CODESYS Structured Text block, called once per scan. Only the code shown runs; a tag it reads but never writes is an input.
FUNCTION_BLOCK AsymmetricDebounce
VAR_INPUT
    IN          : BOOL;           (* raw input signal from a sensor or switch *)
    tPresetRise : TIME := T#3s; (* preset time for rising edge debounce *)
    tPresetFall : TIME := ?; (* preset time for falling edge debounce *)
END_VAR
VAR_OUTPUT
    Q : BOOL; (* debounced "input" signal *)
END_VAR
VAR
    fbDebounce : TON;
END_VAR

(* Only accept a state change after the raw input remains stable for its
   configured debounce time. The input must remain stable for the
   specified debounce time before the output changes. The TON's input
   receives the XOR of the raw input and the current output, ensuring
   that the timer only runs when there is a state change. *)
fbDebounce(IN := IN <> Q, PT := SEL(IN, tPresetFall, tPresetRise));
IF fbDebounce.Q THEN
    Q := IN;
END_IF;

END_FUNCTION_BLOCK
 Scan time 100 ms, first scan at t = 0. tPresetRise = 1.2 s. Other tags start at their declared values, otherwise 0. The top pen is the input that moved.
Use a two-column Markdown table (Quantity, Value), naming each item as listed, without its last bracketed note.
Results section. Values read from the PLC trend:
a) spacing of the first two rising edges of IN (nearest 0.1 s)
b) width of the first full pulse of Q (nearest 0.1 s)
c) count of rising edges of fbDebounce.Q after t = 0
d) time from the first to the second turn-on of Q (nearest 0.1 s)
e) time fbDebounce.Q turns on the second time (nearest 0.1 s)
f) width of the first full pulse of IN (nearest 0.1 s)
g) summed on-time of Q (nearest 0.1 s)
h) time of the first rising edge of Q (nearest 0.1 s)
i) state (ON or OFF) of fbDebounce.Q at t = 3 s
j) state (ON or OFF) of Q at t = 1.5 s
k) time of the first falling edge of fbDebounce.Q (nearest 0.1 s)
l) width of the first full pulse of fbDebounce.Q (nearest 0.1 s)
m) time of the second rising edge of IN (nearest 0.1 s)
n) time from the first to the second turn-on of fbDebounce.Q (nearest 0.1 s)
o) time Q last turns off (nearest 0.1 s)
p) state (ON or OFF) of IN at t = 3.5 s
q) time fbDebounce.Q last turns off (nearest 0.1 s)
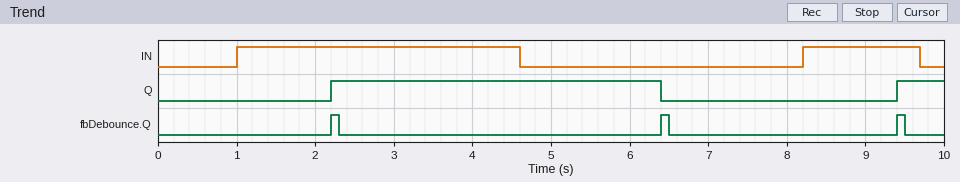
| Quantity | Value |
|---|---|
| spacing of the first two rising edges of IN | 7.2 s |
| width of the first full pulse of Q | 4.2 s |
| count of rising edges of fbDebounce.Q after t = 0 | 3 |
| time from the first to the second turn-on of Q | 7.2 s |
| time fbDebounce.Q turns on the second time | 6.4 s |
| width of the first full pulse of IN | 3.6 s |
| summed on-time of Q | 4.8 s |
| time of the first rising edge of Q | 2.2 s |
| state (ON or OFF) of fbDebounce.Q at t = 3 s | OFF |
| state (ON or OFF) of Q at t = 1.5 s | OFF |
| time of the first falling edge of fbDebounce.Q | 2.3 s |
| width of the first full pulse of fbDebounce.Q | 0.1 s |
| time of the second rising edge of IN | 8.2 s |
| time from the first to the second turn-on of fbDebounce.Q | 4.2 s |
| time Q last turns off | 6.4 s |
| state (ON or OFF) of IN at t = 3.5 s | ON |
| time fbDebounce.Q last turns off | 9.5 s |
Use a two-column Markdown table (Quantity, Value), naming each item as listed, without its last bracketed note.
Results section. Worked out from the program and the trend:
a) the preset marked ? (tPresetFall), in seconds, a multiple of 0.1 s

| Quantity | Value |
|---|---|
| the preset marked ? (tPresetFall), in seconds, a multiple of 0.1 s | 1.8 s |
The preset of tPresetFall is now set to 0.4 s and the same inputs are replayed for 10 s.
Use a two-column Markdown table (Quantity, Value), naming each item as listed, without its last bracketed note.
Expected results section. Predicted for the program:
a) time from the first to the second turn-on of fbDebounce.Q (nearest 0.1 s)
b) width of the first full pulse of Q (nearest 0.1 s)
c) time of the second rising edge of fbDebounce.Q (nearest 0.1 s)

| Quantity | Value |
|---|---|
| time from the first to the second turn-on of fbDebounce.Q | 2.8 s |
| width of the first full pulse of Q | 2.8 s |
| time of the second rising edge of fbDebounce.Q | 5.0 s |
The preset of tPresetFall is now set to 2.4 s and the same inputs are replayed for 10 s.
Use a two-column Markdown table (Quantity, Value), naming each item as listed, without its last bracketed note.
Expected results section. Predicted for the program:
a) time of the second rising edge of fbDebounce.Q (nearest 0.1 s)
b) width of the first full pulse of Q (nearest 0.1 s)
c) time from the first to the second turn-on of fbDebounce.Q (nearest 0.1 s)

| Quantity | Value |
|---|---|
| time of the second rising edge of fbDebounce.Q | 7.0 s |
| width of the first full pulse of Q | 4.8 s |
| time from the first to the second turn-on of fbDebounce.Q | 4.8 s |
